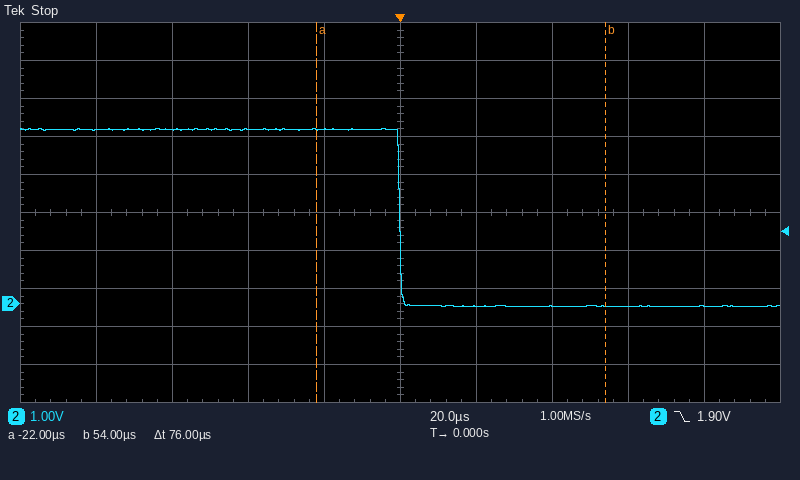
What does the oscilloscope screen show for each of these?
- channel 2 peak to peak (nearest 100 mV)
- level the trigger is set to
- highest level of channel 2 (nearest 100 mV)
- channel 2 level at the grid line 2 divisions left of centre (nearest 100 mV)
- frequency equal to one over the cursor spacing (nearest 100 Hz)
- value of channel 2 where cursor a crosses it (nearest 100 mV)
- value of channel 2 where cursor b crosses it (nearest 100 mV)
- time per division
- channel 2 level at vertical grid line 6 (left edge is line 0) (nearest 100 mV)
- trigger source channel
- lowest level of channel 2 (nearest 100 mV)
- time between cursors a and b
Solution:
4.7 V
1.90 V
4.6 V
4.6 V
13.2 kHz
4.6 V
-100 mV
20 µs
-100 mV
channel 2
-100 mV
76 µs
